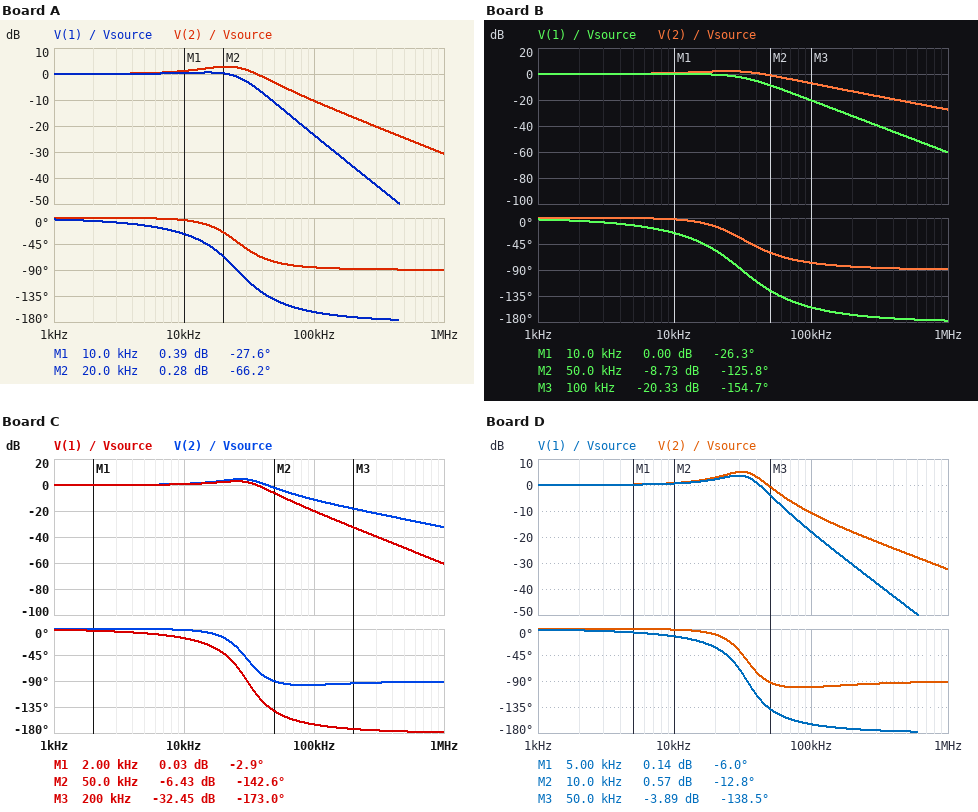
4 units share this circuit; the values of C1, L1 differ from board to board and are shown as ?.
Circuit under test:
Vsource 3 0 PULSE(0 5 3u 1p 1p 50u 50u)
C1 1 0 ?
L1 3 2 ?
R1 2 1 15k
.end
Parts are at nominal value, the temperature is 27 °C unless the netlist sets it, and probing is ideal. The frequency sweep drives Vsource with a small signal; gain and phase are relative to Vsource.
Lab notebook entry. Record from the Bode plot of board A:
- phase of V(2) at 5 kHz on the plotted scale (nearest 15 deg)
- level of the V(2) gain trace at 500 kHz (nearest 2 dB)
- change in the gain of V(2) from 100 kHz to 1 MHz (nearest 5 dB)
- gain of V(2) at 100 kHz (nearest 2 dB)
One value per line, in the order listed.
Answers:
0 deg
-24 dB
-20 dB
-10 dB
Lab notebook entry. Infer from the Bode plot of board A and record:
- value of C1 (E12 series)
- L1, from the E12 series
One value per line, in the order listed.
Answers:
470 pF
82 mH
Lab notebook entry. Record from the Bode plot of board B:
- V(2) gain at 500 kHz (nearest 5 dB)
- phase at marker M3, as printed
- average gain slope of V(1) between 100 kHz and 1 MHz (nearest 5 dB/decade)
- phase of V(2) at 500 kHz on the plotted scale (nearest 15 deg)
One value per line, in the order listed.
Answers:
-20 dB
-154.7 deg
-40 dB/decade
-90 deg
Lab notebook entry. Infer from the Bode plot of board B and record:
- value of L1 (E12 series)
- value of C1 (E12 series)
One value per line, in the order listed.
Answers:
56 mH
470 pF
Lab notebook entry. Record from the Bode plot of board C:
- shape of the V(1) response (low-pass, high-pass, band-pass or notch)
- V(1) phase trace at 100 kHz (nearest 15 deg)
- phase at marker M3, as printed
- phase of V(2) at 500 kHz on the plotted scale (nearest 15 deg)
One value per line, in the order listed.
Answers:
low-pass
-165 deg
-173.0 deg
-90 deg
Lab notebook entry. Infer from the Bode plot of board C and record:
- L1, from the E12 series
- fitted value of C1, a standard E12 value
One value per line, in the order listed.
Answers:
100 mH
270 pF
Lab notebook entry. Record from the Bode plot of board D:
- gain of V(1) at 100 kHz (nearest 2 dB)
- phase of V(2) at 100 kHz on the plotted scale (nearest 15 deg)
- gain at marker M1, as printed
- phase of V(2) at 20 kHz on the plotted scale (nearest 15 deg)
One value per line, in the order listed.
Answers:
-18 dB
-105 deg
0.14 dB
-15 deg
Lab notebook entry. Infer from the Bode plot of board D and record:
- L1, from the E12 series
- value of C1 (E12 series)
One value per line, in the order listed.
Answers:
100 mH
220 pF
